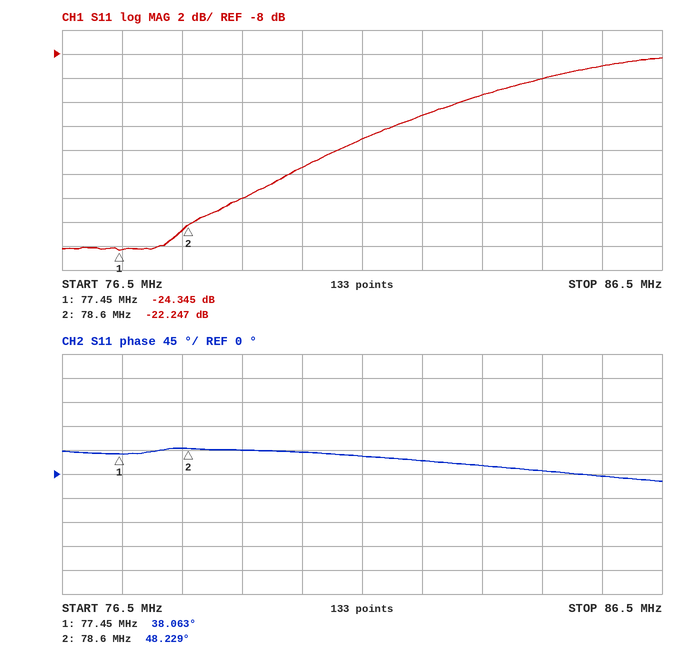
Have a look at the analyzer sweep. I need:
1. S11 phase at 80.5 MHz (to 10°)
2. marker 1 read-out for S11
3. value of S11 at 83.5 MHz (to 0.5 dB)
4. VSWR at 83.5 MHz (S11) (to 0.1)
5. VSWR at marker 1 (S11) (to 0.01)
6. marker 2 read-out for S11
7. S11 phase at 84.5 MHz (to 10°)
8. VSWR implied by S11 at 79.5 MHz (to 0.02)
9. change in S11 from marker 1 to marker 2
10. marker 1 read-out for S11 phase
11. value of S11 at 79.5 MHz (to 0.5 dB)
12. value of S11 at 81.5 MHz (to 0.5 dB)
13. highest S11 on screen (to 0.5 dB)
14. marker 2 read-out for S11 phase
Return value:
40°
-24.345 dB
-11.5 dB
1.7
1.13
-22.247 dB
10°
1.22
2.098 dB
38.063°
-20.0 dB
-15.0 dB
-8.5 dB
48.229°
